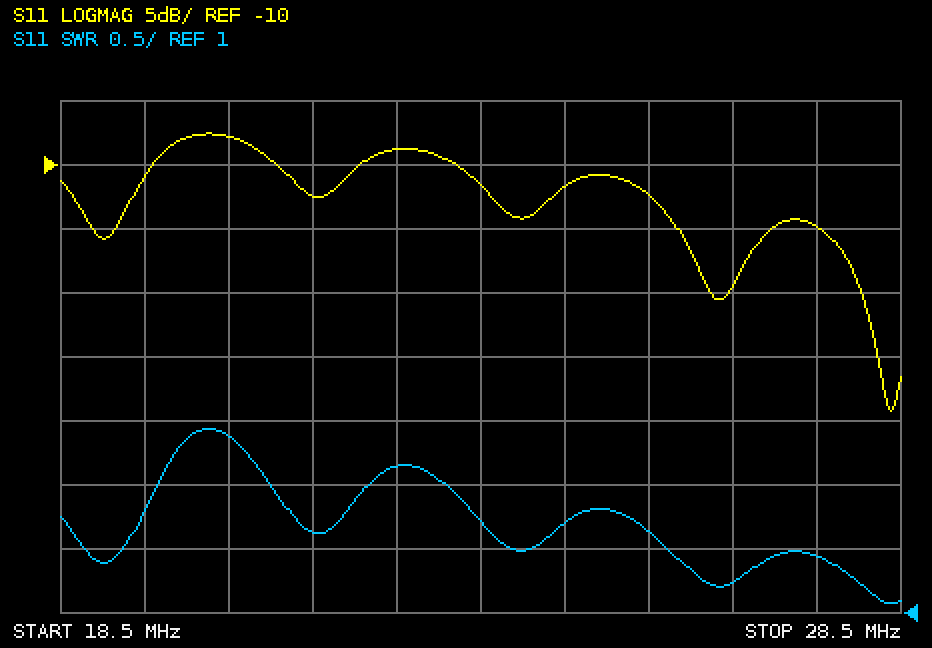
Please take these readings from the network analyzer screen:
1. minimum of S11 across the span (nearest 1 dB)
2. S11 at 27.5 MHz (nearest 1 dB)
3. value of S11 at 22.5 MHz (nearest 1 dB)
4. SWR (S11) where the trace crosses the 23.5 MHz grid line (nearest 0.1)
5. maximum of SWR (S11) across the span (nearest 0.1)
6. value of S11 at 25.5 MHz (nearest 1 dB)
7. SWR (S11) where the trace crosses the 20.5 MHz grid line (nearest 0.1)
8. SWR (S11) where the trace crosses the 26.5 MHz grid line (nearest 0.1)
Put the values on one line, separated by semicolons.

-29 dB; -15 dB; -9 dB; 1.7; 2.4; -12 dB; 2.4; 1.2
